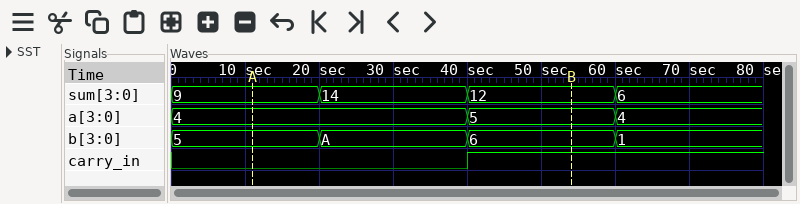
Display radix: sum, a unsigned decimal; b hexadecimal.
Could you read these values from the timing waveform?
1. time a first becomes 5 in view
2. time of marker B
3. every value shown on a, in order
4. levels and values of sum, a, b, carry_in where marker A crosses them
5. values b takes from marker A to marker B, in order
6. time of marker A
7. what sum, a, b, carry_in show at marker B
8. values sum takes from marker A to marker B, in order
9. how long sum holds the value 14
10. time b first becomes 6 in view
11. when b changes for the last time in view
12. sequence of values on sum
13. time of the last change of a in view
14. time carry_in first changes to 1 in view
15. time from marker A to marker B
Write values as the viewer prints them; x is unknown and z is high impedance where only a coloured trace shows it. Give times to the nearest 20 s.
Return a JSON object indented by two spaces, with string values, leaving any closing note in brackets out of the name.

{
  "time a first becomes 5 in view": "40 s",
  "time of marker B": "60 s",
  "every value shown on a, in order": "4, 5, 4",
  "levels and values of sum, a, b, carry_in where marker A crosses them": "sum=9, a=4, b=5, carry_in=0",
  "values b takes from marker A to marker B, in order": "5, A, 6",
  "time of marker A": "20 s",
  "what sum, a, b, carry_in show at marker B": "sum=12, a=5, b=6, carry_in=1",
  "values sum takes from marker A to marker B, in order": "9, 14, 12",
  "how long sum holds the value 14": "20 s",
  "time b first becomes 6 in view": "40 s",
  "when b changes for the last time in view": "60 s",
  "sequence of values on sum": "9, 14, 12, 6",
  "time of the last change of a in view": "60 s",
  "time carry_in first changes to 1 in view": "40 s",
  "time from marker A to marker B": "40 s"
}
